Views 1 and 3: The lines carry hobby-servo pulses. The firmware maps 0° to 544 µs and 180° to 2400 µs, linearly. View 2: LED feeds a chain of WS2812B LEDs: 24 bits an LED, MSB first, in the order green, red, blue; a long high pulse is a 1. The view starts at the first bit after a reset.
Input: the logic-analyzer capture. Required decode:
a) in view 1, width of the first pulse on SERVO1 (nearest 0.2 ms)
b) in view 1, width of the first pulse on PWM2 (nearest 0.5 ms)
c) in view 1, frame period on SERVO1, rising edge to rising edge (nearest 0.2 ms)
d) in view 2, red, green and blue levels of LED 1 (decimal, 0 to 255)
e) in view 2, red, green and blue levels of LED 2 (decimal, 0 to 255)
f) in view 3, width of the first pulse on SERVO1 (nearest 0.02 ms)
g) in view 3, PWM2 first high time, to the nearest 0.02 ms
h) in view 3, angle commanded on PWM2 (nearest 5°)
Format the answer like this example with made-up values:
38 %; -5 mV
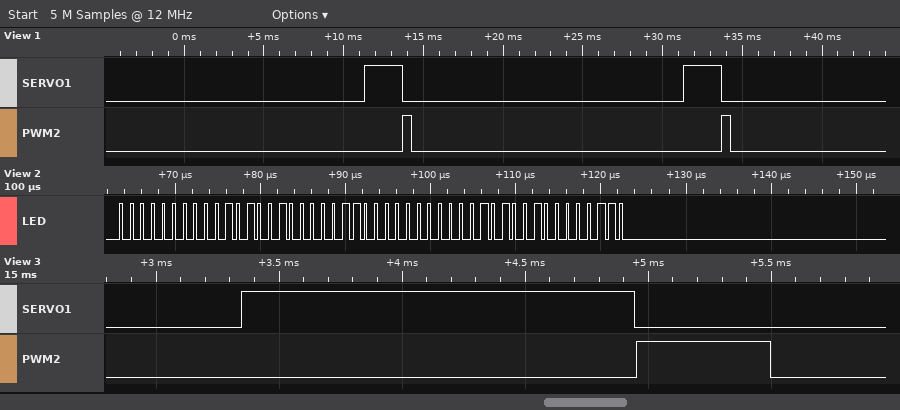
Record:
2.4 ms; 0.5 ms; 20.0 ms; 41, 0, 6; 41, 0, 6; 1.60 ms; 0.54 ms; 0°
